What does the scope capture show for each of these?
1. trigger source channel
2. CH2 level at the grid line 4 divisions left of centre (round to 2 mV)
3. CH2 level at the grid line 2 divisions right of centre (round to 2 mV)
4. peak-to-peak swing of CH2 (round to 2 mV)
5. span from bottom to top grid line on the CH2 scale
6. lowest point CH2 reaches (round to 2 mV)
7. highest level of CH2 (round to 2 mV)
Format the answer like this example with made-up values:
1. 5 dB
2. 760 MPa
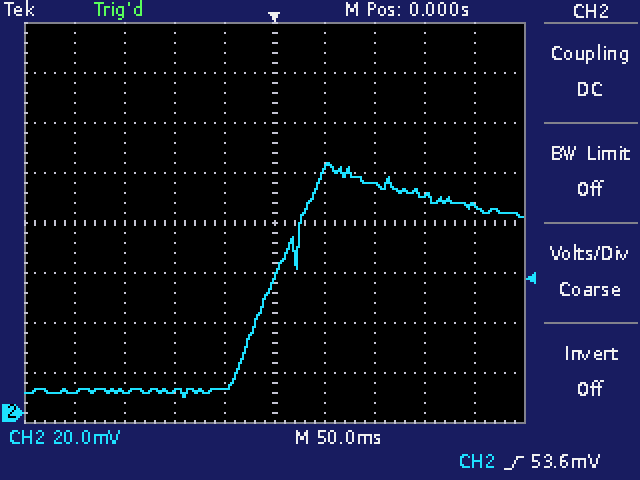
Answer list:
1. CH2
2. 8 mV
3. 92 mV
4. 94 mV
5. 160 mV
6. 6 mV
7. 100 mV
